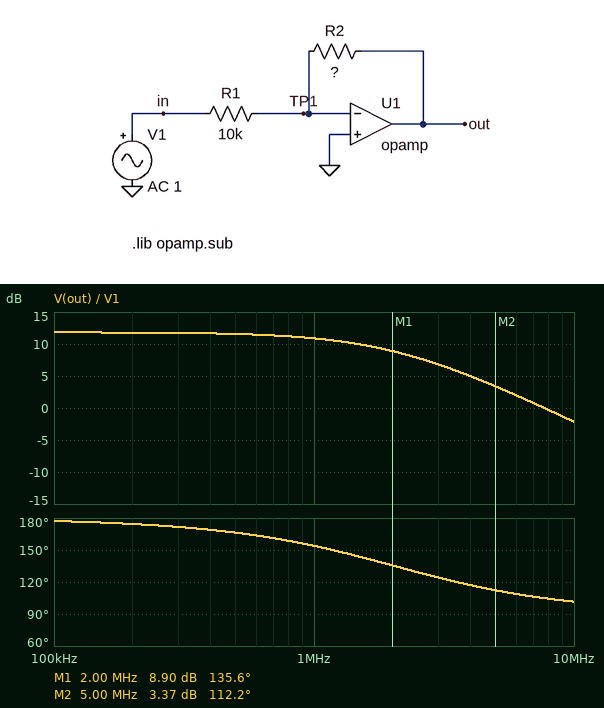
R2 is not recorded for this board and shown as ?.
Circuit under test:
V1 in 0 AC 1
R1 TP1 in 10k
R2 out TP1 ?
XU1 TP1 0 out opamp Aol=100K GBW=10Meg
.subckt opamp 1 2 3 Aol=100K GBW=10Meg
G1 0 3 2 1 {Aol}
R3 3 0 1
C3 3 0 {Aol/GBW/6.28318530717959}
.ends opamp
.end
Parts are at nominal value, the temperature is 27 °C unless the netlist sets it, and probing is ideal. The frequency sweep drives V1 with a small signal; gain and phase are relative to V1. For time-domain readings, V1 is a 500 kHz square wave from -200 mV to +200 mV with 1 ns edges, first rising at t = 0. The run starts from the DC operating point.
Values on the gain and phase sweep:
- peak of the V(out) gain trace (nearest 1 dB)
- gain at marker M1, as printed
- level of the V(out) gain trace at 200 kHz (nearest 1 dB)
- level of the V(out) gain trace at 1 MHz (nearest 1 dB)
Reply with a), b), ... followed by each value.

a) 12 dB
b) 8.90 dB
c) 12 dB
d) 11 dB
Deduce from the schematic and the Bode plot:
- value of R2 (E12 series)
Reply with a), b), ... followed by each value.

a) 39 kΩ
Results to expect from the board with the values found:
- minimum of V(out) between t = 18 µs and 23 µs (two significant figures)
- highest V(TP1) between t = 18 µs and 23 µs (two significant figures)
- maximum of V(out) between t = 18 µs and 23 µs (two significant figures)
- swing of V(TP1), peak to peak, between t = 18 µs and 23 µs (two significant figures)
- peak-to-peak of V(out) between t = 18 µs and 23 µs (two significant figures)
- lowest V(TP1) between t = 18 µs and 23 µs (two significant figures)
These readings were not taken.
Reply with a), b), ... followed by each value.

a) -780 mV
b) 320 mV
c) 780 mV
d) 630 mV
e) 1.6 V
f) -320 mV
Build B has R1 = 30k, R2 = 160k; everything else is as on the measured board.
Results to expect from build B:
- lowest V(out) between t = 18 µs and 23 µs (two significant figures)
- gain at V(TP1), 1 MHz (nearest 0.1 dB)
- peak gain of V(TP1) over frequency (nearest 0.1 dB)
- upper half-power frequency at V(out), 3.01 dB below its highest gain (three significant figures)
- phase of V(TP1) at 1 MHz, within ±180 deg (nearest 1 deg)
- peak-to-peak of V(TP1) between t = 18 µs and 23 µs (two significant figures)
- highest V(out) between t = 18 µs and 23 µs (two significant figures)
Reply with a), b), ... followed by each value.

a) -1.1 V
b) -6.9 dB
c) -1.5 dB
d) 1.58 MHz
e) 58 deg
f) 670 mV
g) 1.1 V
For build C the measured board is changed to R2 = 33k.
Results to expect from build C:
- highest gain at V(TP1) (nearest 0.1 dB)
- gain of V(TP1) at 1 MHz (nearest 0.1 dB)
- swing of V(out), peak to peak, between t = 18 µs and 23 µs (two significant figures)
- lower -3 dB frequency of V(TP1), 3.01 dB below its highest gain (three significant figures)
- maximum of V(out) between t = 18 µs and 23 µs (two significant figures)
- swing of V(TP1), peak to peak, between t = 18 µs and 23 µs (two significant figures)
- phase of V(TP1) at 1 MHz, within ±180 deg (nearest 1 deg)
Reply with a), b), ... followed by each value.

a) -2.3 dB
b) -10.4 dB
c) 1.3 V
d) 2.33 MHz
e) 660 mV
f) 610 mV
g) 67 deg
